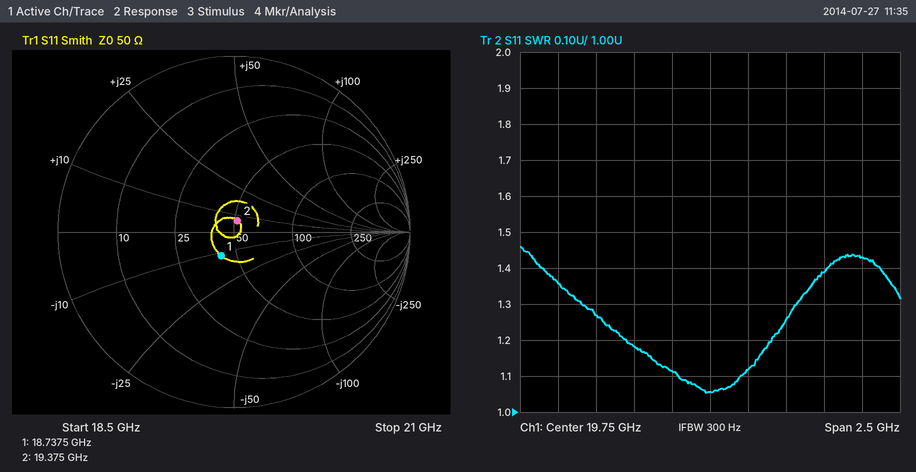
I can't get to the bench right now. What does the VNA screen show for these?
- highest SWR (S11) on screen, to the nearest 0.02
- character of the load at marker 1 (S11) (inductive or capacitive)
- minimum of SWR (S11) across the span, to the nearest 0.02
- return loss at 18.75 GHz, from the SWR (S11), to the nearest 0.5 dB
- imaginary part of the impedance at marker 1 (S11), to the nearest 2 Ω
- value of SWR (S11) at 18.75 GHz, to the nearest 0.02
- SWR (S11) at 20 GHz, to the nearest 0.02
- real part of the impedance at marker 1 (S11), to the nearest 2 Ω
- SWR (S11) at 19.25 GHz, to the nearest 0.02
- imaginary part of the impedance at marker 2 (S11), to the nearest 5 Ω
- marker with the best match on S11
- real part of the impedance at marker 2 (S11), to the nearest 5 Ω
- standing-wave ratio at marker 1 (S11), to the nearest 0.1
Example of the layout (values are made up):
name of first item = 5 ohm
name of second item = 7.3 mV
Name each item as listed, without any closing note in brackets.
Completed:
highest SWR (S11) on screen, to the nearest 0.02 = 1.46
character of the load at marker 1 (S11) = capacitive
minimum of SWR (S11) across the span, to the nearest 0.02 = 1.06
return loss at 18.75 GHz, from the SWR (S11), to the nearest 0.5 dB = 16.5 dB
imaginary part of the impedance at marker 1 (S11), to the nearest 2 Ω = -12 Ω
value of SWR (S11) at 18.75 GHz, to the nearest 0.02 = 1.36
SWR (S11) at 20 GHz, to the nearest 0.02 = 1.12
real part of the impedance at marker 1 (S11), to the nearest 2 Ω = 42 Ω
SWR (S11) at 19.25 GHz, to the nearest 0.02 = 1.18
imaginary part of the impedance at marker 2 (S11), to the nearest 5 Ω = +5 Ω
marker with the best match on S11 = marker 2
real part of the impedance at marker 2 (S11), to the nearest 5 Ω = 50 Ω
standing-wave ratio at marker 1 (S11), to the nearest 0.1 = 1.4
